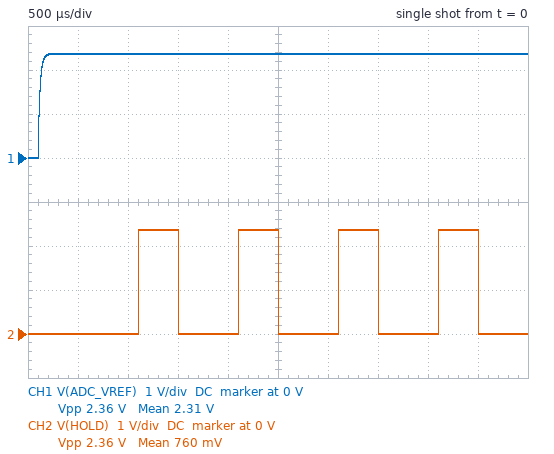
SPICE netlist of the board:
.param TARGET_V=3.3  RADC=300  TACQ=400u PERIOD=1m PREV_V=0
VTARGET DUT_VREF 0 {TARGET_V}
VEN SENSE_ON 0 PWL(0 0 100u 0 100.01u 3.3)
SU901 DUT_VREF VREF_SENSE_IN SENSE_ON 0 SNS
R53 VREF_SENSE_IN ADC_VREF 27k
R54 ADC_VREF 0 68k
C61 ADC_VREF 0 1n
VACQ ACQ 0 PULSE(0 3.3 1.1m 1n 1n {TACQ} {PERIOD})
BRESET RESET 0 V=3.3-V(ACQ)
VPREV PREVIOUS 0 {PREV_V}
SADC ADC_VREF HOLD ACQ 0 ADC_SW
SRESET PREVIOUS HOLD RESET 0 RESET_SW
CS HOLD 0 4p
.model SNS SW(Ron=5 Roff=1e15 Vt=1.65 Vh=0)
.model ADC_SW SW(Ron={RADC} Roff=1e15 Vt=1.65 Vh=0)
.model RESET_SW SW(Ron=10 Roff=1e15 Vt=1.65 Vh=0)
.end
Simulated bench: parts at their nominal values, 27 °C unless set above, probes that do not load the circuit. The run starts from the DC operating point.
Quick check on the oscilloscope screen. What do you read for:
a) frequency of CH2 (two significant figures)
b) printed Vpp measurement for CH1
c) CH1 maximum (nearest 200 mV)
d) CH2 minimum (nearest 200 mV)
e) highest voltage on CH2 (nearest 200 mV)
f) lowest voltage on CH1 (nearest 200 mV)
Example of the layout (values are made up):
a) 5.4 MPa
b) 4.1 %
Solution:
a) 1.0 kHz
b) 2.36 V
c) 2.4 V
d) 0 V
e) 2.4 V
f) 0 V
